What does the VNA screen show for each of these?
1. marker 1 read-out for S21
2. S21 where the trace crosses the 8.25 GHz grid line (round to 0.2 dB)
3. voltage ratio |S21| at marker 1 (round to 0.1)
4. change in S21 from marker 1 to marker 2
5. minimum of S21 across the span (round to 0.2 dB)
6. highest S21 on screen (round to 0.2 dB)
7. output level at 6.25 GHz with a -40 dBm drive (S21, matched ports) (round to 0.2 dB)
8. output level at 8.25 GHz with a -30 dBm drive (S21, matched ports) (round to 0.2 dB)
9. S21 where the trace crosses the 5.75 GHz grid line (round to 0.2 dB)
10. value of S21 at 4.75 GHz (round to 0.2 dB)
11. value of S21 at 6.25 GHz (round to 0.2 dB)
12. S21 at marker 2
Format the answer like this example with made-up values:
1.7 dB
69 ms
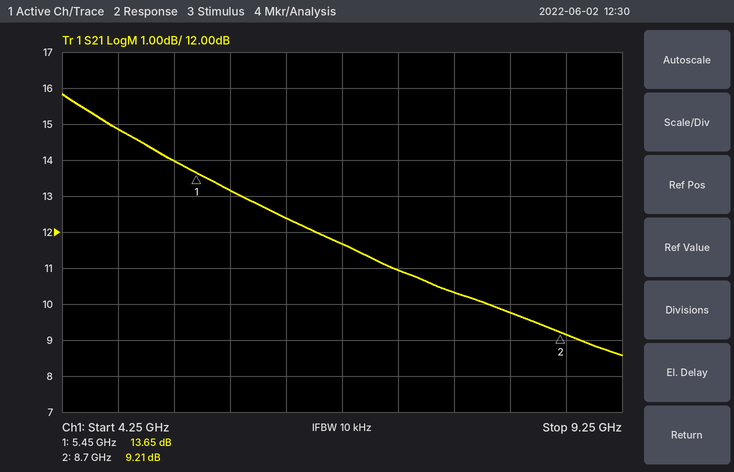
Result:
13.65 dB
9.8 dB
4.8
-4.44 dB
8.6 dB
15.8 dB
-27.6 dBm
-20.2 dBm
13.2 dB
14.8 dB
12.4 dB
9.21 dB
